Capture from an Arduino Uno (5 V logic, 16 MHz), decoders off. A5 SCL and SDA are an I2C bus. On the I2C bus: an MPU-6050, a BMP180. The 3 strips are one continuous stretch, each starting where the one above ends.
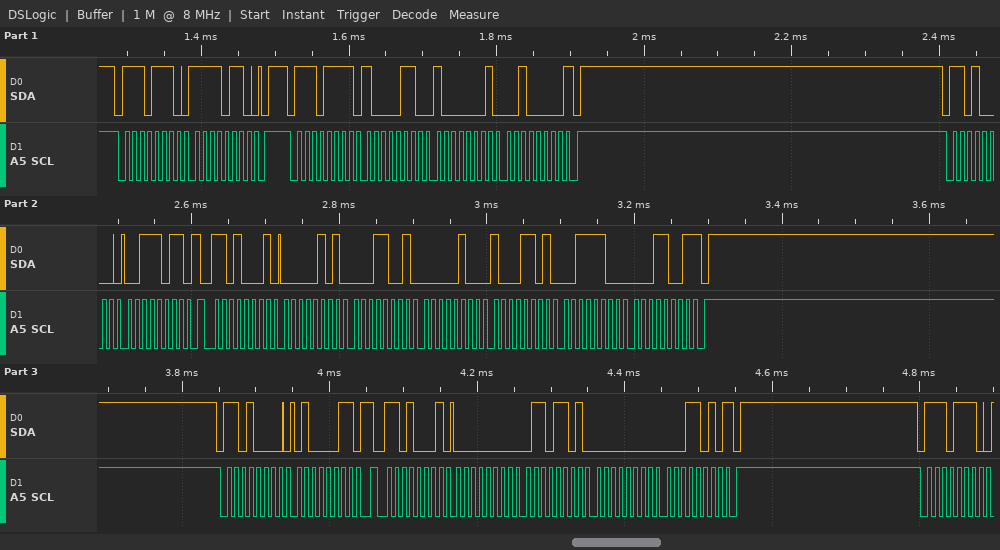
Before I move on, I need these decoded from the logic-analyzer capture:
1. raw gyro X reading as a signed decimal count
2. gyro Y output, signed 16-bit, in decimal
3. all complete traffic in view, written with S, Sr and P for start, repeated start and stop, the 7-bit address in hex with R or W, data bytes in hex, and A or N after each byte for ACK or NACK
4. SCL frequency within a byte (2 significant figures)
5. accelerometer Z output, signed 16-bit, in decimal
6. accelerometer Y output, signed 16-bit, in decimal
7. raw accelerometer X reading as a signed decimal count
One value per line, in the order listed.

109
26
S 77W A F6 A P S 77R A 86 A 81 A 20 N P S 68W A 3B A Sr 68R A 05 A 19 A 04 A 8D A 3C A 19 N P S 68W A 43 A Sr 68R A 00 A 6D A 00 A 1A N P S 77W A
100 kHz
15385
1165
1305
